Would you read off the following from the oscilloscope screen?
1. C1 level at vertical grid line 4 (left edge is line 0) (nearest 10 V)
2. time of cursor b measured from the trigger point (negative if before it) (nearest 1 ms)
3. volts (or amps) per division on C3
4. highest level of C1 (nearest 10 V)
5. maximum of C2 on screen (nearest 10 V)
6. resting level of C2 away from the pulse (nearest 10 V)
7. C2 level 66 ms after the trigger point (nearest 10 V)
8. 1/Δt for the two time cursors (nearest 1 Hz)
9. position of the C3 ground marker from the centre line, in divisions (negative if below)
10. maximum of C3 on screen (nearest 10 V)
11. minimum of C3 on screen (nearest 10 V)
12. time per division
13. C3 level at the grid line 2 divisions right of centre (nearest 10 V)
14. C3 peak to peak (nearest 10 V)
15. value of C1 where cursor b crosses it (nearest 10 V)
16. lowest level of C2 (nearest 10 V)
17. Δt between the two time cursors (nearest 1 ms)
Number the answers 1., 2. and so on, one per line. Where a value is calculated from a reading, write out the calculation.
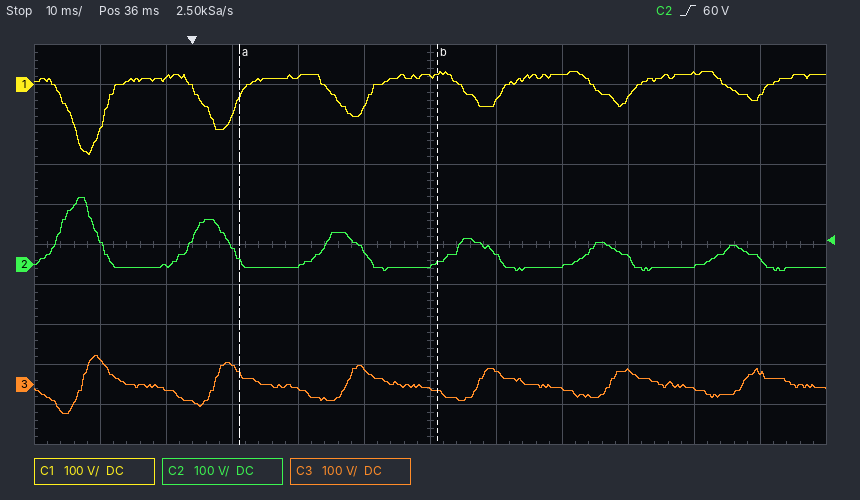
1. 20 V
2. +37 ms
3. 100 V
4. 30 V
5. 170 V
6. -10 V
7. 20 V
8. 1 / 30 ms ≈ 33 Hz
9. -3.5 div
10. 70 V
11. -70 V
12. 10 ms
13. -10 V
14. 70 V − (-70 V) = 140 V
15. 30 V
16. -20 V
17. 30 ms
